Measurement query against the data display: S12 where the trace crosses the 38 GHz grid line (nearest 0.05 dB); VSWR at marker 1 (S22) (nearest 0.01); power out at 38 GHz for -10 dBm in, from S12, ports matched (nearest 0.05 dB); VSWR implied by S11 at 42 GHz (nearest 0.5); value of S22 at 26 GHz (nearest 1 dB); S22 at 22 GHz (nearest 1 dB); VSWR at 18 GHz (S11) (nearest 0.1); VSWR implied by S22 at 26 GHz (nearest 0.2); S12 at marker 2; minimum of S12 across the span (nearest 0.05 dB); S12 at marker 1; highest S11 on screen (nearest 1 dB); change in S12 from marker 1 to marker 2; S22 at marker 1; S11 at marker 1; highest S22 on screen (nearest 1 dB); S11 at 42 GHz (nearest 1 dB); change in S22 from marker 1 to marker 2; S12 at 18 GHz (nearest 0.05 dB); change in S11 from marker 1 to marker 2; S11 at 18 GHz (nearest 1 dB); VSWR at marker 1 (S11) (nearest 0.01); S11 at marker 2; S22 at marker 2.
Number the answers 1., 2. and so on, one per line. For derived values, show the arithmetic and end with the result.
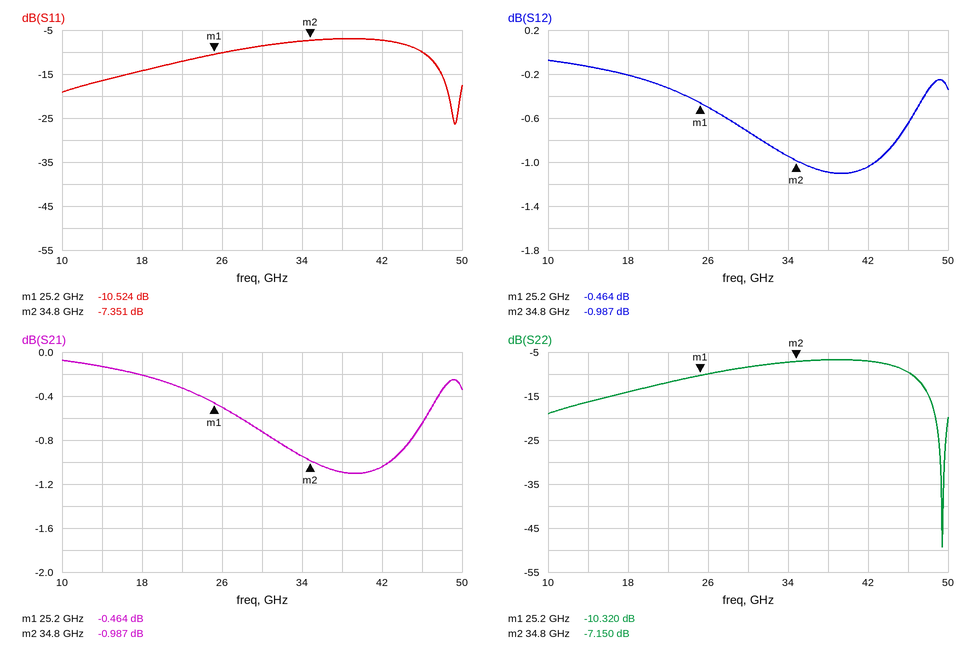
1. -1.10 dB
2. (1 + 0.3048)/(1 − 0.3048) ≈ 1.88
3. -10 dBm + (-1.10 dB) = -11.10 dBm
4. |Γ| = 10^(-7/20) = 0.4467; VSWR = (1 + 0.4467)/(1 − 0.4467) ≈ 2.61, so 2.5 to the nearest 0.5
5. -10 dB
6. -12 dB
7. |Γ| = 10^(-14/20) = 0.1995; VSWR = (1 + 0.1995)/(1 − 0.1995) ≈ 1.5
8. |Γ| = 10^(-10/20) = 0.3162; VSWR = (1 + 0.3162)/(1 − 0.3162) ≈ 1.92, so 2.0 to the nearest 0.2
9. -0.987 dB
10. -1.10 dB
11. -0.464 dB
12. -7 dB
13. -0.987 − (-0.464) = -0.523 dB
14. -10.320 dB
15. -10.524 dB
16. -7 dB
17. -7 dB
18. -7.15 − (-10.32) = 3.170 dB
19. -0.20 dB
20. -7.351 − (-10.524) = 3.173 dB
21. -14 dB
22. (1 + 0.2977)/(1 − 0.2977) ≈ 1.85
23. -7.351 dB
24. -7.150 dB
